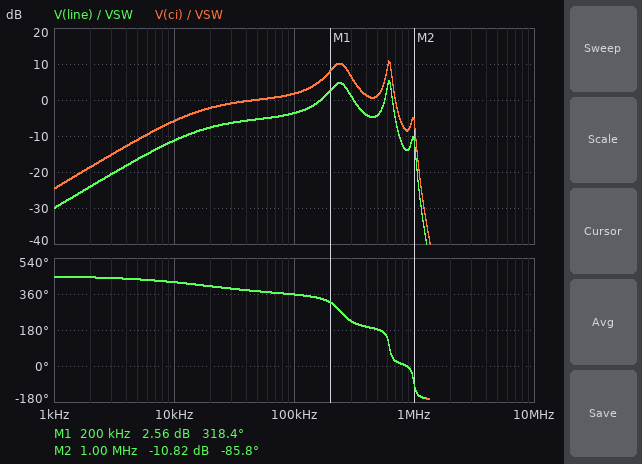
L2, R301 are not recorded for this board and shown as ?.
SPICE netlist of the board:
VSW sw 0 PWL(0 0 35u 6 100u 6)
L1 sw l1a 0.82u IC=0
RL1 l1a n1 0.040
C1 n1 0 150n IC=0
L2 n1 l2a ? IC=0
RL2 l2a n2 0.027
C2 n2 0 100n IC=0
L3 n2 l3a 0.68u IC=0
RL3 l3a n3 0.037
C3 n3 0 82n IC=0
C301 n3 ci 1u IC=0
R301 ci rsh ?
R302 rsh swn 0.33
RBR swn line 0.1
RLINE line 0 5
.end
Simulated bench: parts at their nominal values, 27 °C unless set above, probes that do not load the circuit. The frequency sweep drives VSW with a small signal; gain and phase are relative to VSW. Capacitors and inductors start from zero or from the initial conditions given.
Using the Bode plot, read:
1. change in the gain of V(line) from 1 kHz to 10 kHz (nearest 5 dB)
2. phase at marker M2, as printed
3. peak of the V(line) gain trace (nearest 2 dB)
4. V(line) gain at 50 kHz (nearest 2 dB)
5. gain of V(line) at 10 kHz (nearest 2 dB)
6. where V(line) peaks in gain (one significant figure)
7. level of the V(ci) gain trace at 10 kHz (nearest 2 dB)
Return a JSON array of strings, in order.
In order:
["20 dB", "-85.8 deg", "6 dB", "-6 dB", "-12 dB", "600 kHz", "-6 dB"]
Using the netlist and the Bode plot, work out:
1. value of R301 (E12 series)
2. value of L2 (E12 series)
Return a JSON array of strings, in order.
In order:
["3.9 Ω", "1 µH"]
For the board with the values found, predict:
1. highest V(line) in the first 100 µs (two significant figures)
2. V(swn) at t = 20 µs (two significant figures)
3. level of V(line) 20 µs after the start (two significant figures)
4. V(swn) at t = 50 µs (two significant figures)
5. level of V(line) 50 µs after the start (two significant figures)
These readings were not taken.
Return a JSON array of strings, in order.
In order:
["840 mV", "770 mV", "760 mV", "170 mV", "170 mV"]
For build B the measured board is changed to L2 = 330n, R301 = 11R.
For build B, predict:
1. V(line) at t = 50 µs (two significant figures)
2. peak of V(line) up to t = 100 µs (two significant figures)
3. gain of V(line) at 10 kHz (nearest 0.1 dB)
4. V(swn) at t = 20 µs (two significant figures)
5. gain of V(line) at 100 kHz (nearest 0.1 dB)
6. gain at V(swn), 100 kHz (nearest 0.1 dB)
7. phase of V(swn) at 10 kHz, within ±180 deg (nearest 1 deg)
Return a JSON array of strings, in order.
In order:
["310 mV", "760 mV", "-13.2 dB", "610 mV", "-9.0 dB", "-8.8 dB", "44 deg"]
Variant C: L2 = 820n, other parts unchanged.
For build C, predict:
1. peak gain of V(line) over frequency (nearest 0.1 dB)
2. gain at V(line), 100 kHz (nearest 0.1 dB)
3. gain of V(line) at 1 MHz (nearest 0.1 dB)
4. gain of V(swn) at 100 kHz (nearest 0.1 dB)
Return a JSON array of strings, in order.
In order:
["5.1 dB", "-3.8 dB", "-9.1 dB", "-3.6 dB"]
